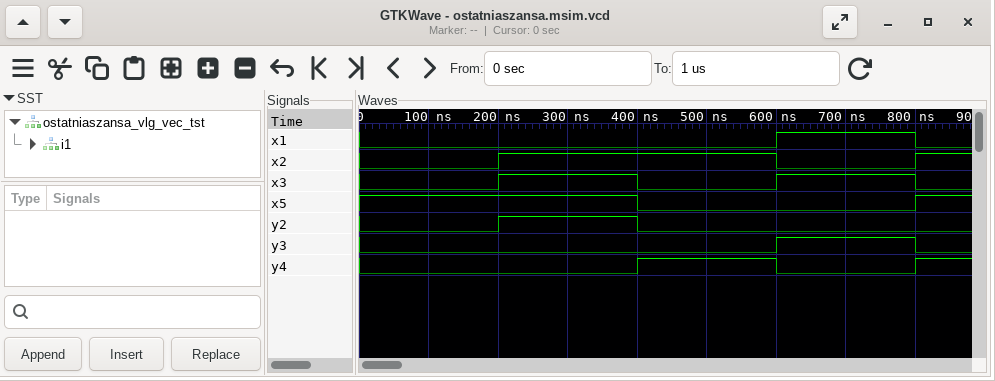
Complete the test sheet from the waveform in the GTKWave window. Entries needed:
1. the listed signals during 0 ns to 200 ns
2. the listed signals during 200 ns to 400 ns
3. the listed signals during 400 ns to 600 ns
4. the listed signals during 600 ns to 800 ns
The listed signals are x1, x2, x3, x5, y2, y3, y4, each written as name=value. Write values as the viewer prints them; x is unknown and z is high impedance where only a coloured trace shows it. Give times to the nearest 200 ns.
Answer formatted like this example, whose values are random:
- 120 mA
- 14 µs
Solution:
- x1=0, x2=0, x3=0, x5=1, y2=0, y3=0, y4=0
- x1=0, x2=1, x3=1, x5=1, y2=1, y3=0, y4=0
- x1=0, x2=1, x3=0, x5=0, y2=0, y3=0, y4=1
- x1=1, x2=0, x3=1, x5=0, y2=0, y3=1, y4=0
